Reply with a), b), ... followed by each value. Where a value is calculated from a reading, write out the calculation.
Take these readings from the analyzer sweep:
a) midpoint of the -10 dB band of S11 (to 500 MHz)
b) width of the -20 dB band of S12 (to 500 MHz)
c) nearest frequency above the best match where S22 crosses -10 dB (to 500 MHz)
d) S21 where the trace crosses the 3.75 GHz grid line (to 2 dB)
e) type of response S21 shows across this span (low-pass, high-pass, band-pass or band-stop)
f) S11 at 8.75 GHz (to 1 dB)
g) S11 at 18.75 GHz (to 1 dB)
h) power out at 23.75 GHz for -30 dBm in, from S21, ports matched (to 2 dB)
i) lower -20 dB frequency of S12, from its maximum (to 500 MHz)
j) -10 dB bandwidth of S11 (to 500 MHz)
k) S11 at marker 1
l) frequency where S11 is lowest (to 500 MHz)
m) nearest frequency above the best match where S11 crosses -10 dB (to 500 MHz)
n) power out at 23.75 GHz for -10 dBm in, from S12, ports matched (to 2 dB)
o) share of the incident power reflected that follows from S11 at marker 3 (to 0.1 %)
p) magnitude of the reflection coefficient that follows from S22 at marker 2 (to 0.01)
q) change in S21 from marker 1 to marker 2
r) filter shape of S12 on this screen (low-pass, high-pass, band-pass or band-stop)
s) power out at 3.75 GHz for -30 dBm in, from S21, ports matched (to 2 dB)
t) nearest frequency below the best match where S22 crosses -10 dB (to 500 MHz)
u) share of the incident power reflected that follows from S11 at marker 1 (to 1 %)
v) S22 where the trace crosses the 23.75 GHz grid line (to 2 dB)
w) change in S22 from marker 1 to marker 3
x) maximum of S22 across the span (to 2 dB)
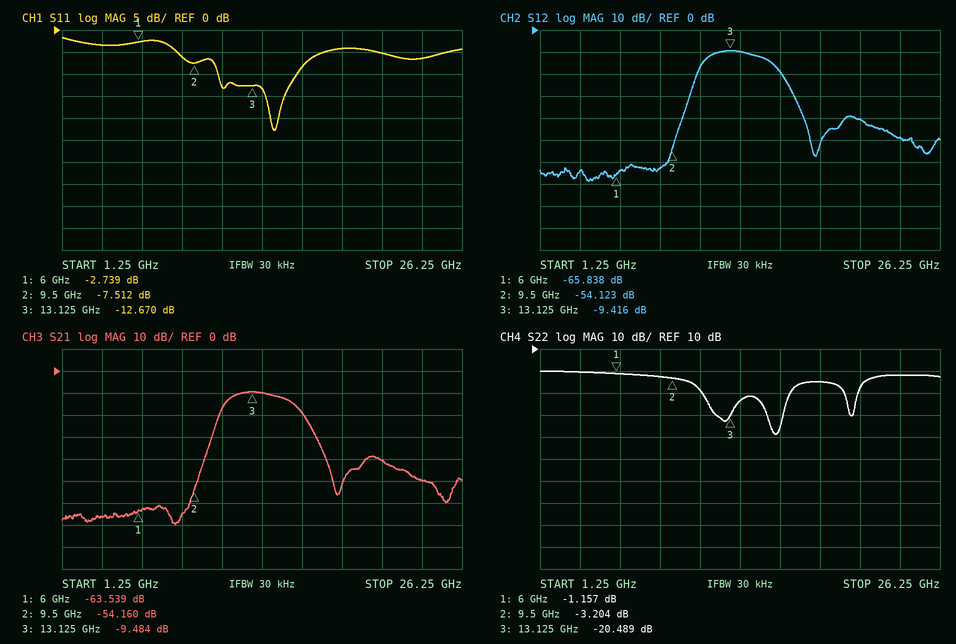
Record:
a) 13.5 GHz
b) 17.0 GHz − 10.5 GHz = 6.5 GHz
c) 17.0 GHz
d) -66 dB
e) band-pass
f) -6 dB
g) -4 dB
h) -30 dBm + (-50 dB) = -80 dBm
i) 10.5 GHz
j) 16.0 GHz − 11.0 GHz = 5.0 GHz
k) -2.739 dB
l) 14.5 GHz
m) 16.0 GHz
n) -10 dBm + (-48 dB) = -58 dBm
o) 10^(-12.67/10) ≈ 5.4 %
p) 10^(-3.204/20) ≈ 0.69
q) -54.16 − (-63.539) = 9.379 dB
r) band-pass
s) -30 dBm + (-66 dB) = -96 dBm
t) 11.5 GHz
u) 10^(-2.739/10) ≈ 53 %
v) -2 dB
w) -20.489 − (-1.157) = -19.332 dB
x) 0 dB
